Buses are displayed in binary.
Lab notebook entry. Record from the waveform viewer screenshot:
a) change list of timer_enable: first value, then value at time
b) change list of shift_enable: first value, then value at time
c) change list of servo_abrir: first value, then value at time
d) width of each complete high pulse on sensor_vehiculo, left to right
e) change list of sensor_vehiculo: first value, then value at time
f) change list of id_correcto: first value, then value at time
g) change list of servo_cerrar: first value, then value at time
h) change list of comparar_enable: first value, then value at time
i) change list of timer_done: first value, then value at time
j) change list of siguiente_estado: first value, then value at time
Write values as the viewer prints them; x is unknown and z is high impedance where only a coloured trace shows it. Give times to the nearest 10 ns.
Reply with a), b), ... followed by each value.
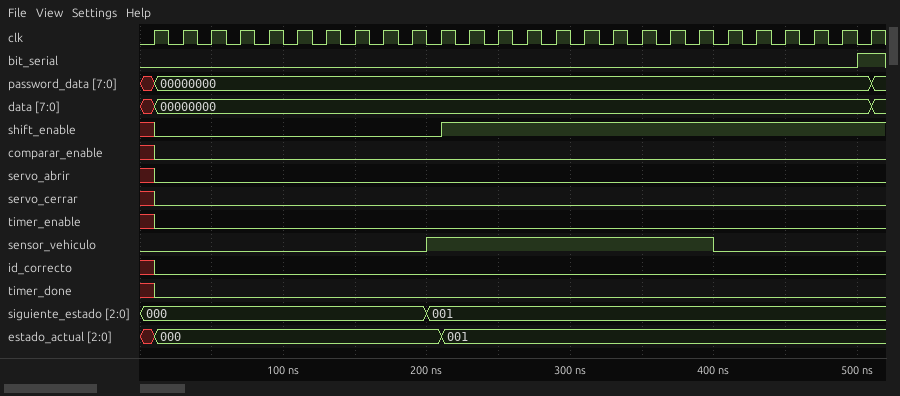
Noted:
a) x, 0 at 10 ns
b) x, 0 at 10 ns, 1 at 210 ns
c) x, 0 at 10 ns
d) 200 ns
e) 0, 1 at 200 ns, 0 at 400 ns
f) x, 0 at 10 ns
g) x, 0 at 10 ns
h) x, 0 at 10 ns
i) x, 0 at 10 ns
j) 000, 001 at 200 ns
